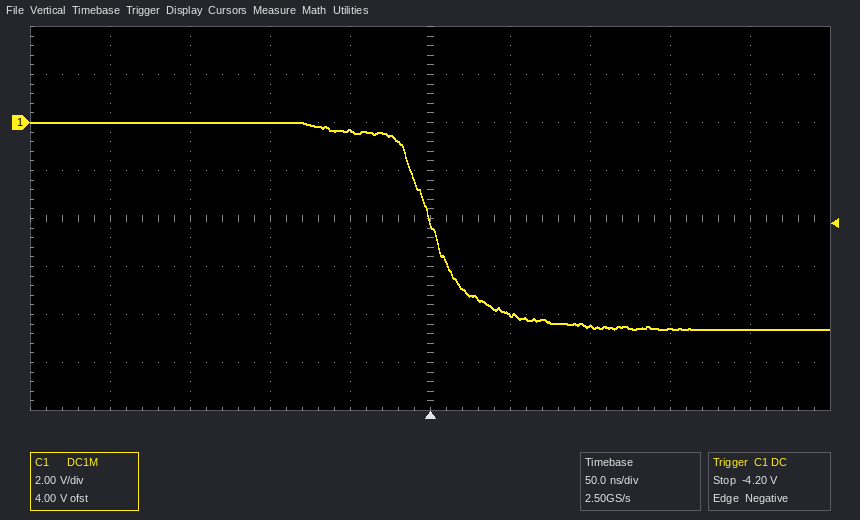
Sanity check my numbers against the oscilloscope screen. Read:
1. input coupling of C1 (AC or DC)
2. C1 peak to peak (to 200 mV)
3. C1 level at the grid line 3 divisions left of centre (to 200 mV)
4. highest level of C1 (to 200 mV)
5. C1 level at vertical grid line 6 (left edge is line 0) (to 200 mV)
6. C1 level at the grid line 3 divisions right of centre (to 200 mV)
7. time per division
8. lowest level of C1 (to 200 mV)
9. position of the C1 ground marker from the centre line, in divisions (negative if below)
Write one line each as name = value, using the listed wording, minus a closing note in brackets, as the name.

input coupling of C1 = DC
C1 peak to peak = 8.6 V
C1 level at the grid line 3 divisions left of centre = 0.0 V
highest level of C1 = 0.0 V
C1 level at vertical grid line 6 (left edge is line 0) = -8.0 V
C1 level at the grid line 3 divisions right of centre = -8.6 V
time per division = 50 ns
lowest level of C1 = -8.6 V
position of the C1 ground marker from the centre line, in divisions = +2.0 div
